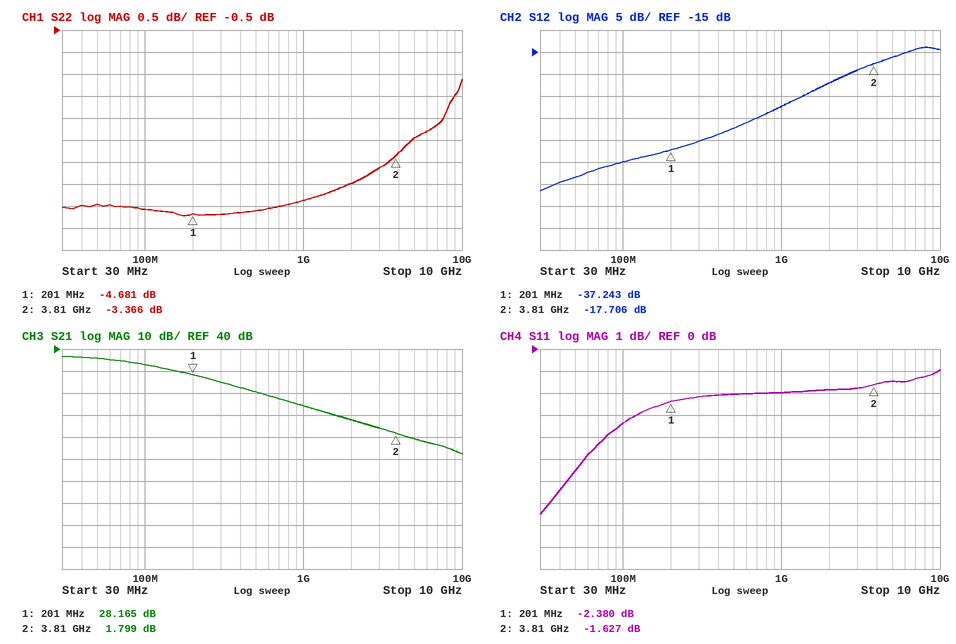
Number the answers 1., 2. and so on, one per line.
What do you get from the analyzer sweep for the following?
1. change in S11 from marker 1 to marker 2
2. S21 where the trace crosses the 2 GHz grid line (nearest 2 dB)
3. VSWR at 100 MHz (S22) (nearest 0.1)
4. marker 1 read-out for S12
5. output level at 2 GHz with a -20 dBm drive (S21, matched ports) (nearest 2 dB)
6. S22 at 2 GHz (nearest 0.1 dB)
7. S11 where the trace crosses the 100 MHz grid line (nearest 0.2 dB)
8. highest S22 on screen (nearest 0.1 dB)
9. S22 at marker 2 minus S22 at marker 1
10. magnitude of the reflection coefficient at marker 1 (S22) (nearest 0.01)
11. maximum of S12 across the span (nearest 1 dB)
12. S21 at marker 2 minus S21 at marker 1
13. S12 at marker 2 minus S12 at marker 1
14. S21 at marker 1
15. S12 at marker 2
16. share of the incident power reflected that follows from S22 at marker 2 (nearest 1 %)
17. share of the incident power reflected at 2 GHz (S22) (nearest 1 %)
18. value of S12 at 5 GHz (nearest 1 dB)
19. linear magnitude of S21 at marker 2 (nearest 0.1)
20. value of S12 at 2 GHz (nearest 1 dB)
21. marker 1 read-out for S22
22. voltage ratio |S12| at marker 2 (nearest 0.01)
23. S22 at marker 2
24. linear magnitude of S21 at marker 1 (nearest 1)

1. 0.753 dB
2. 8 dB
3. 3.9
4. -37.243 dB
5. -12 dBm
6. -4.0 dB
7. -3.4 dB
8. -1.6 dB
9. 1.315 dB
10. 0.58
11. -14 dB
12. -26.366 dB
13. 19.537 dB
14. 28.165 dB
15. -17.706 dB
16. 46 %
17. 40 %
18. -16 dB
19. 1.2
20. -22 dB
21. -4.681 dB
22. 0.13
23. -3.366 dB
24. 26
